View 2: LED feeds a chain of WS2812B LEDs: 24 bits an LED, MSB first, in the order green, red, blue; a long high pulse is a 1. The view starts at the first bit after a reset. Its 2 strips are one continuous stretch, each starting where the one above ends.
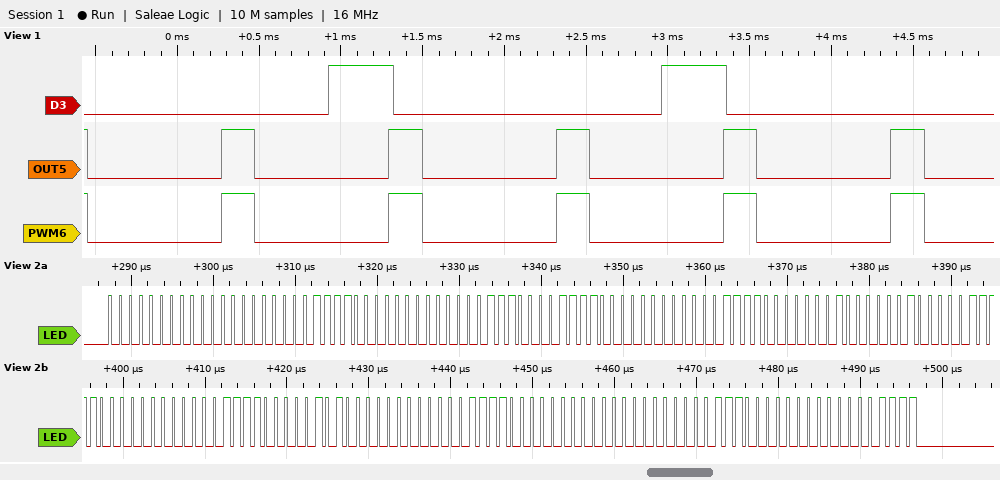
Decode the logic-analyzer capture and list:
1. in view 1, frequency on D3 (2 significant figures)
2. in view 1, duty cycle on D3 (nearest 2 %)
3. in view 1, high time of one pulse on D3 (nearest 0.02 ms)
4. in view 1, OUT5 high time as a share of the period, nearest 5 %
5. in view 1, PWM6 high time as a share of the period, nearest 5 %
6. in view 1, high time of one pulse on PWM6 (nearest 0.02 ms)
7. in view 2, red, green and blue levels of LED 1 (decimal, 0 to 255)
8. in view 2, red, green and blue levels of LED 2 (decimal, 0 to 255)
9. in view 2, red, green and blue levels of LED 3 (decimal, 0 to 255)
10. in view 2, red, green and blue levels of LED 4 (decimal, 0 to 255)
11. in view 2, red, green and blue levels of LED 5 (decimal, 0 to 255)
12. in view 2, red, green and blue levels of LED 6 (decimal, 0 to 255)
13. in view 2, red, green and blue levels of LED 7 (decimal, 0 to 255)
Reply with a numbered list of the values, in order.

1. 490 Hz
2. 20 %
3. 0.40 ms
4. 20 %
5. 20 %
6. 0.20 ms
7. 0, 0, 15
8. 7, 0, 15
9. 15, 0, 1
10. 15, 2, 0
11. 5, 15, 0
12. 0, 15, 0
13. 0, 14, 15
